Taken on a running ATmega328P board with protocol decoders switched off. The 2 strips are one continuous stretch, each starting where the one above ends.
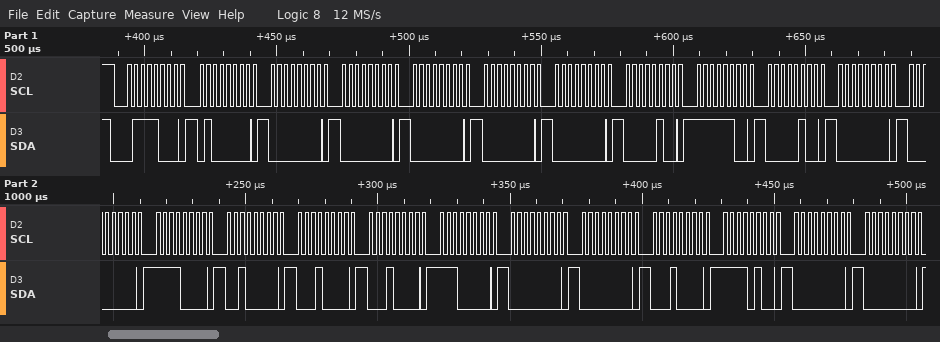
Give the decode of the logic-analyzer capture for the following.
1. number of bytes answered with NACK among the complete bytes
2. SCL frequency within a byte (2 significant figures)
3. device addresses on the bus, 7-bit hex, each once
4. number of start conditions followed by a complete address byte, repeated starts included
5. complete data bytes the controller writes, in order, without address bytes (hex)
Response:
0
400 kHz
0x3C
1
40 00 00 00 00 00 04 FC 04 00 00 F0 20 10 10 E0 00 00 10 F4 00 00
